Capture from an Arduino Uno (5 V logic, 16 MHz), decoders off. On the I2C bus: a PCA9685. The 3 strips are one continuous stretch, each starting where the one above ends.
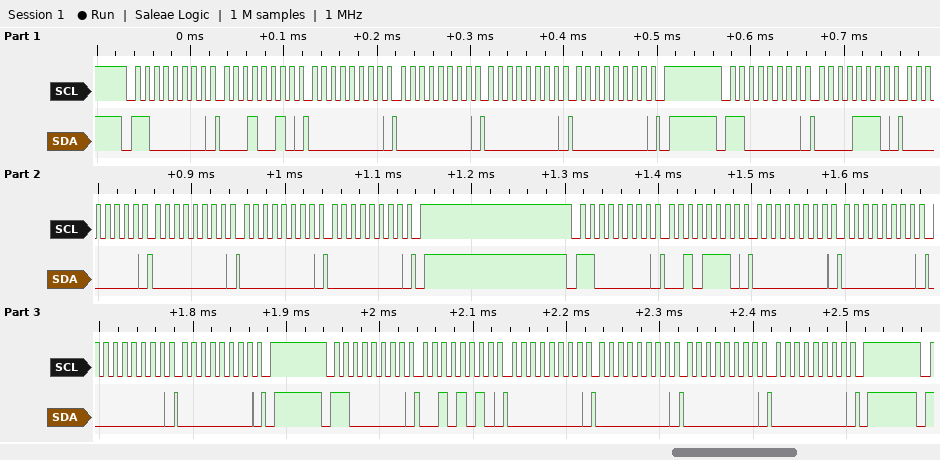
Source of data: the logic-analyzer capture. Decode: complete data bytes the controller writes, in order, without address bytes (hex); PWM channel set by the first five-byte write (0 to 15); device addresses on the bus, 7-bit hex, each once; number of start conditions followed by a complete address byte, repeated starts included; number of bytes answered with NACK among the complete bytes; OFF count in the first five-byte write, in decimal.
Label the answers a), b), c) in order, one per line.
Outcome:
a) 12 00 00 00 00 0E 00 00 00 00 2E 00 00 00 00 2A 00 00 00 00
b) 3
c) 0x60
d) 4
e) 0
f) 0
